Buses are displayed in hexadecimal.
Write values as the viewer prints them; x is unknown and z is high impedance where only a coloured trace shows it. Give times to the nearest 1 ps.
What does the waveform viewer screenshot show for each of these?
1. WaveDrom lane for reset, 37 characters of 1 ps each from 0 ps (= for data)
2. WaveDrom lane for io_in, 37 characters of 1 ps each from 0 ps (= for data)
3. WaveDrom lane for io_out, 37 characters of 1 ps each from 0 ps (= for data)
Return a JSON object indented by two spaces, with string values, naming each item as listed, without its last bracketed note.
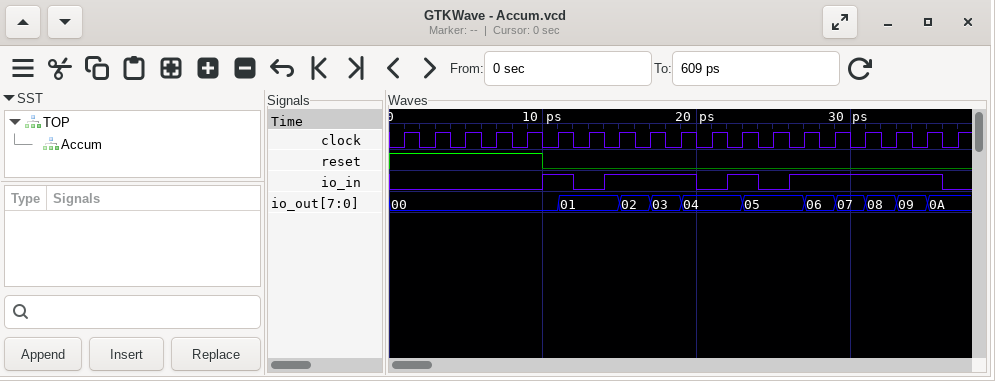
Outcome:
{
  "WaveDrom lane for reset, 37 characters of 1 ps each from 0 ps": "{name: 'reset', wave: '1.........0..........................'}",
  "WaveDrom lane for io_in, 37 characters of 1 ps each from 0 ps": "{name: 'io_in', wave: '0.........1.0.1.....0.1.0.1.........0'}",
  "WaveDrom lane for io_out, 37 characters of 1 ps each from 0 ps": "{name: 'io_out', wave: '=..........=...=.=.=...=...=.=.=.=.=.', data: '00 01 02 03 04 05 06 07 08 09 0A'}"
}
